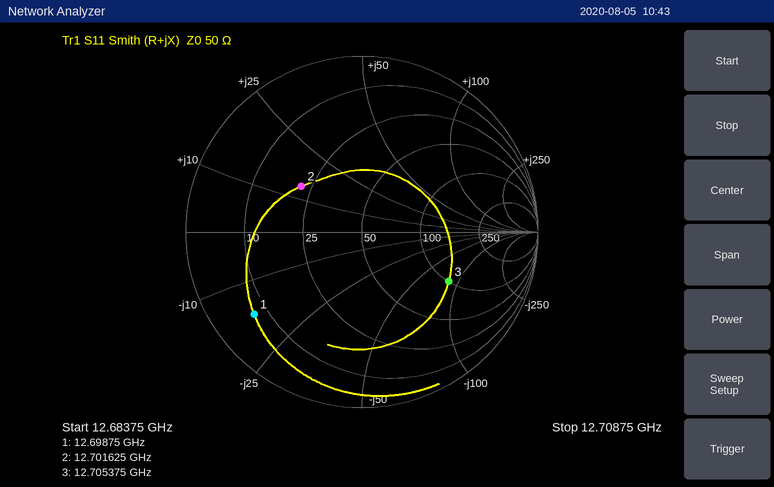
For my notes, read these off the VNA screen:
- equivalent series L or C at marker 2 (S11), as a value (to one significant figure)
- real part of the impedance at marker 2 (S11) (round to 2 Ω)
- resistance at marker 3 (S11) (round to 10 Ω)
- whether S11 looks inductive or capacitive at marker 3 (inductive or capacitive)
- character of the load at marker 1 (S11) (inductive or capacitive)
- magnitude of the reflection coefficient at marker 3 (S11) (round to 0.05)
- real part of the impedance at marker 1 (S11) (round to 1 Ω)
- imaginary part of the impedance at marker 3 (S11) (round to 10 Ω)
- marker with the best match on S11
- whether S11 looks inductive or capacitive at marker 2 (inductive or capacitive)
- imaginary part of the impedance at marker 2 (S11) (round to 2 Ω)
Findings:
200 pH
22 Ω
100 Ω
capacitive
capacitive
0.55
7 Ω
-80 Ω
marker 2
inductive
+14 Ω
